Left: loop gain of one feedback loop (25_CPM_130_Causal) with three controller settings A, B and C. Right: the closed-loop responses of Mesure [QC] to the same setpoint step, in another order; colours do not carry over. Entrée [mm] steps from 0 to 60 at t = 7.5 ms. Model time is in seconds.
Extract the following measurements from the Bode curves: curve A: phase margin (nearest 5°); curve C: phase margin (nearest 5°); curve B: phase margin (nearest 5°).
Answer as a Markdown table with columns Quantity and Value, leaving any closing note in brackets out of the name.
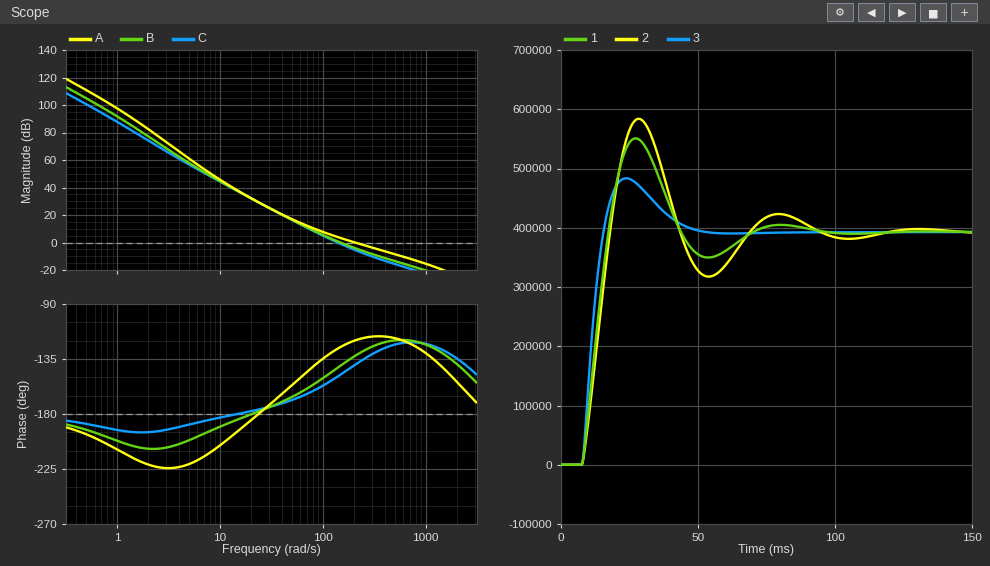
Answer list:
| Quantity | Value |
|---|---|
| curve A: phase margin | 60° |
| curve C: phase margin | 30° |
| curve B: phase margin | 40° |
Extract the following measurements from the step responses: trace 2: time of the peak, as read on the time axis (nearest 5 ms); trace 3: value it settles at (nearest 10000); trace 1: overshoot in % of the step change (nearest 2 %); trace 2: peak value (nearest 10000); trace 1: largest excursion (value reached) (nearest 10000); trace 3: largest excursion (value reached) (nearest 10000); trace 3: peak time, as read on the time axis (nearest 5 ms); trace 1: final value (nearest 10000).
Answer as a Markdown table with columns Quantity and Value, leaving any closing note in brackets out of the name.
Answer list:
| Quantity | Value |
|---|---|
| trace 2: time of the peak, as read on the time axis | 30 ms |
| trace 3: value it settles at | 390000 |
| trace 1: overshoot in % of the step change | 40 % |
| trace 2: peak value | 580000 |
| trace 1: largest excursion (value reached) | 550000 |
| trace 3: largest excursion (value reached) | 480000 |
| trace 3: peak time, as read on the time axis | 25 ms |
| trace 1: final value | 390000 |
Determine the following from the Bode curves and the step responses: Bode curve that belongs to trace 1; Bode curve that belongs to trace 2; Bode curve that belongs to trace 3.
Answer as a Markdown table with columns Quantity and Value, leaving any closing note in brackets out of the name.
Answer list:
| Quantity | Value |
|---|---|
| Bode curve that belongs to trace 1 | B |
| Bode curve that belongs to trace 2 | C |
| Bode curve that belongs to trace 3 | A |
